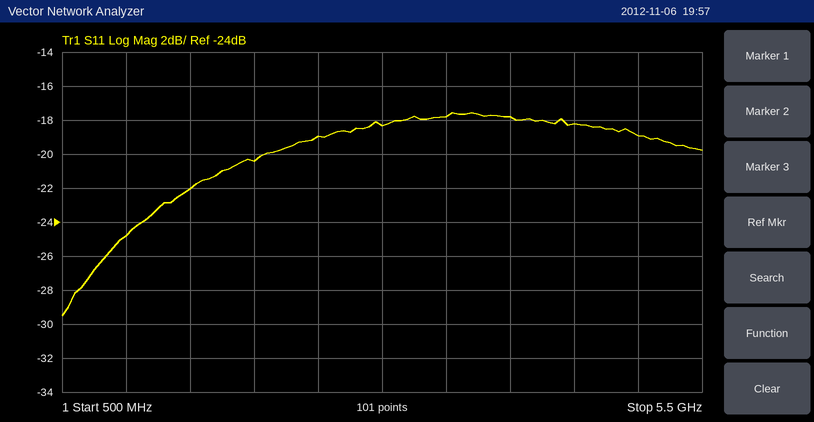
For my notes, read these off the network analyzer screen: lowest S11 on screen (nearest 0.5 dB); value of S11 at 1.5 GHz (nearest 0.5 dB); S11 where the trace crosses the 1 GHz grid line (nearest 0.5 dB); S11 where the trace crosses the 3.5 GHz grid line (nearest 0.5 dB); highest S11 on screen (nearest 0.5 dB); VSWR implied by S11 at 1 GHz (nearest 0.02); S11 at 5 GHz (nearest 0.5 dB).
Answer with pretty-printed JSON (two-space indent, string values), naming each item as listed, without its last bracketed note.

{
  "lowest S11 on screen": "-29.5 dB",
  "value of S11 at 1.5 GHz": "-22.0 dB",
  "S11 where the trace crosses the 1 GHz grid line": "-25.0 dB",
  "S11 where the trace crosses the 3.5 GHz grid line": "-18.0 dB",
  "highest S11 on screen": "-17.5 dB",
  "VSWR implied by S11 at 1 GHz": "1.12",
  "S11 at 5 GHz": "-19.0 dB"
}
